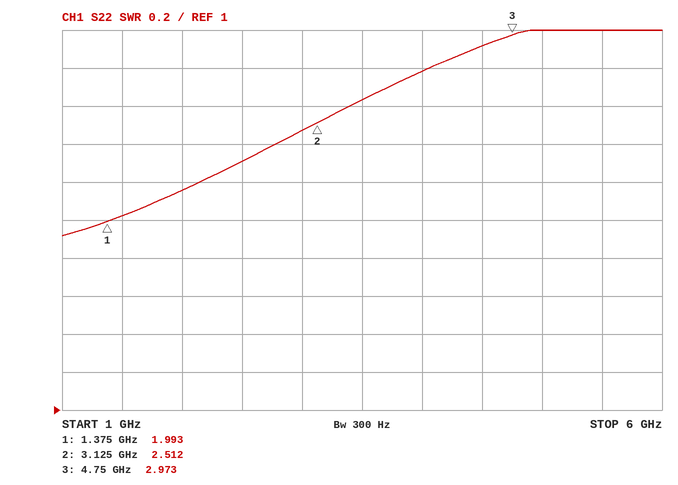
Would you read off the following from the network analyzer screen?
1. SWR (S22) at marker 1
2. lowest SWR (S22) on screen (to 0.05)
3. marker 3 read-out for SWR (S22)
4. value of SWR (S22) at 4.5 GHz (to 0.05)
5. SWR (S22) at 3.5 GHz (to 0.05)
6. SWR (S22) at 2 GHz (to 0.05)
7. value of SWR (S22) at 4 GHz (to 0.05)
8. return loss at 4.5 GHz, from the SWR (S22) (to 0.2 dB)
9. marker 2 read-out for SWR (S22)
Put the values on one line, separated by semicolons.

1.993; 1.90; 2.973; 2.90; 2.65; 2.15; 2.80; 6.2 dB; 2.512
